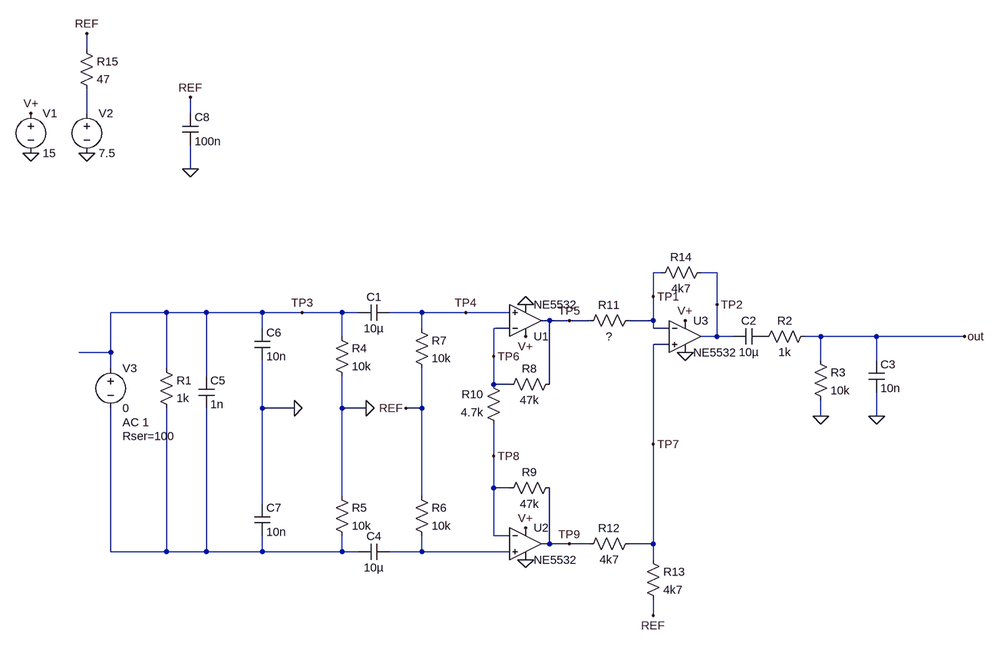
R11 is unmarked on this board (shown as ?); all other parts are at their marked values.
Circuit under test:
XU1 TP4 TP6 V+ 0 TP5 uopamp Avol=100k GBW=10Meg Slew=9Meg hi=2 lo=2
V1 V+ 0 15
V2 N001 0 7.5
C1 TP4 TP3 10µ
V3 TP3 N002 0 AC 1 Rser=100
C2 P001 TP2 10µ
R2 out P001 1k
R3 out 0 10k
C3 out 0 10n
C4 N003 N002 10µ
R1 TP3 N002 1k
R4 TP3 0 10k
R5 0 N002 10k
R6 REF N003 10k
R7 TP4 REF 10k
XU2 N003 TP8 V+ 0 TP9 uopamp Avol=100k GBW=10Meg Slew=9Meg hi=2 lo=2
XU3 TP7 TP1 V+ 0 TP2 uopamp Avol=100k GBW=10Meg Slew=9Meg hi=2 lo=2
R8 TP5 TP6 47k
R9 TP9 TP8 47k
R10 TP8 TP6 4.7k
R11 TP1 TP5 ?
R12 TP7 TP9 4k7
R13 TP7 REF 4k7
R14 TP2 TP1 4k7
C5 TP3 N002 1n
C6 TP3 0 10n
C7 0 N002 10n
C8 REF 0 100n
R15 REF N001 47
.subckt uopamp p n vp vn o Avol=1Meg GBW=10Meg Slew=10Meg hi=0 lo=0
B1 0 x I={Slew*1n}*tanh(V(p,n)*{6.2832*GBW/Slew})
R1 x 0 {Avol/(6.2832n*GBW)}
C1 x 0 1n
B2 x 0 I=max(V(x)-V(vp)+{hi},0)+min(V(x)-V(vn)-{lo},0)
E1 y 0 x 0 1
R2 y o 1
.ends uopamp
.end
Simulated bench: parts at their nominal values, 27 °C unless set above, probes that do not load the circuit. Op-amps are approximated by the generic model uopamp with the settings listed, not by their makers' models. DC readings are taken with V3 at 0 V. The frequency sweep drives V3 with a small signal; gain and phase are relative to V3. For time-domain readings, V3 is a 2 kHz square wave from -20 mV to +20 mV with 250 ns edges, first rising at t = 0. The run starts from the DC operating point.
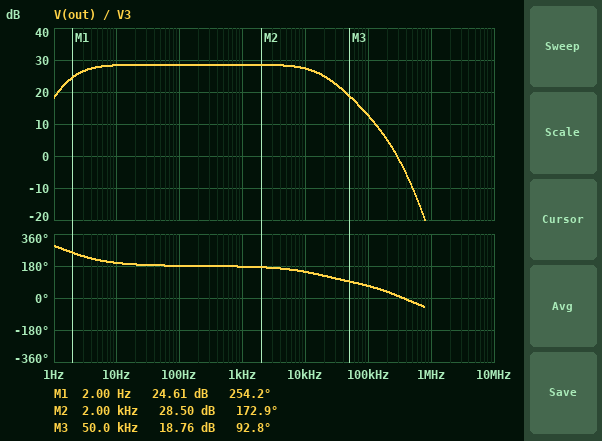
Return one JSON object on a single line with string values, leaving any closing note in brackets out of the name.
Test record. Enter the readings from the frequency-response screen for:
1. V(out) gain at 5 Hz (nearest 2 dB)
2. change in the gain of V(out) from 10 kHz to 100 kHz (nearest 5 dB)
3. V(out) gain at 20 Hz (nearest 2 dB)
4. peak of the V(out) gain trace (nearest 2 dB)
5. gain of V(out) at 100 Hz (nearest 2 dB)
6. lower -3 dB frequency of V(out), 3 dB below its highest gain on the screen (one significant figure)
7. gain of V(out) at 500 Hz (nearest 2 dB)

{"V(out) gain at 5 Hz": "28 dB", "change in the gain of V(out) from 10 kHz to 100 kHz": "-15 dB", "V(out) gain at 20 Hz": "28 dB", "peak of the V(out) gain trace": "28 dB", "gain of V(out) at 100 Hz": "28 dB", "lower -3 dB frequency of V(out), 3 dB below its highest gain on the screen": "2 Hz", "gain of V(out) at 500 Hz": "28 dB"}
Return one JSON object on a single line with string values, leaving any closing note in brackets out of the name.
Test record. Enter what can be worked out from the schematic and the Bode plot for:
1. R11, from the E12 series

{"R11, from the E12 series": "2.7 kΩ"}
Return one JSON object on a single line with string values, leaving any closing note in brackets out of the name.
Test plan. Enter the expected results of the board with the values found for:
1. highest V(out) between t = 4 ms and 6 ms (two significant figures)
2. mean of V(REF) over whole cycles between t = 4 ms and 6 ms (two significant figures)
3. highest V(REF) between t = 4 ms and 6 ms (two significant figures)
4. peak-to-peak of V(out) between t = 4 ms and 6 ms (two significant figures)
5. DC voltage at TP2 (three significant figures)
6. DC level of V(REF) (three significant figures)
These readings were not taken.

{"highest V(out) between t = 4 ms and 6 ms": "59 mV", "mean of V(REF) over whole cycles between t = 4 ms and 6 ms": "7.5 V", "highest V(REF) between t = 4 ms and 6 ms": "7.5 V", "peak-to-peak of V(out) between t = 4 ms and 6 ms": "1.1 V", "DC voltage at TP2": "7.50 V", "DC level of V(REF)": "7.50 V"}
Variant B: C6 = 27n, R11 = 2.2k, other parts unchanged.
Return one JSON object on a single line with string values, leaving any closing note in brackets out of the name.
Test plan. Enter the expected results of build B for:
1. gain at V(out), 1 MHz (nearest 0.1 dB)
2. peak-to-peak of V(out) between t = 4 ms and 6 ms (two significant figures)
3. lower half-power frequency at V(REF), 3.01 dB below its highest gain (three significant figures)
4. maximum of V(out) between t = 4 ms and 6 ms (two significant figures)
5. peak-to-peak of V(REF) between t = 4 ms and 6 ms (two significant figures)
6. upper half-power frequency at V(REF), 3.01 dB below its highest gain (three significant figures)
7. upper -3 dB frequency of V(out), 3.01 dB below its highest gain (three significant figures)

{"gain at V(out), 1 MHz": "-26.5 dB", "peak-to-peak of V(out) between t = 4 ms and 6 ms": "1.3 V", "lower half-power frequency at V(REF), 3.01 dB below its highest gain": "1.71 Hz", "maximum of V(out) between t = 4 ms and 6 ms": "69 mV", "peak-to-peak of V(REF) between t = 4 ms and 6 ms": "2.0 mV", "upper half-power frequency at V(REF), 3.01 dB below its highest gain": "34.3 kHz", "upper -3 dB frequency of V(out), 3.01 dB below its highest gain": "17.2 kHz"}
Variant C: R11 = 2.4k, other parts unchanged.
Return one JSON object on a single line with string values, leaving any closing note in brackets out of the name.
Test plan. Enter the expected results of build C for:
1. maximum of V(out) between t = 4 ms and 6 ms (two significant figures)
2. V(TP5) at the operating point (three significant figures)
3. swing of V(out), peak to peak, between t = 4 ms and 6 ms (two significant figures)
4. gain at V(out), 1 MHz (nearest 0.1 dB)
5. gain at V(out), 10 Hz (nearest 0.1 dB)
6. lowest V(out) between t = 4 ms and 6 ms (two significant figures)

{"maximum of V(out) between t = 4 ms and 6 ms": "65 mV", "V(TP5) at the operating point": "7.50 V", "swing of V(out), peak to peak, between t = 4 ms and 6 ms": "1.2 V", "gain at V(out), 1 MHz": "-24.4 dB", "gain at V(out), 10 Hz": "29.2 dB", "lowest V(out) between t = 4 ms and 6 ms": "-1.1 V"}
